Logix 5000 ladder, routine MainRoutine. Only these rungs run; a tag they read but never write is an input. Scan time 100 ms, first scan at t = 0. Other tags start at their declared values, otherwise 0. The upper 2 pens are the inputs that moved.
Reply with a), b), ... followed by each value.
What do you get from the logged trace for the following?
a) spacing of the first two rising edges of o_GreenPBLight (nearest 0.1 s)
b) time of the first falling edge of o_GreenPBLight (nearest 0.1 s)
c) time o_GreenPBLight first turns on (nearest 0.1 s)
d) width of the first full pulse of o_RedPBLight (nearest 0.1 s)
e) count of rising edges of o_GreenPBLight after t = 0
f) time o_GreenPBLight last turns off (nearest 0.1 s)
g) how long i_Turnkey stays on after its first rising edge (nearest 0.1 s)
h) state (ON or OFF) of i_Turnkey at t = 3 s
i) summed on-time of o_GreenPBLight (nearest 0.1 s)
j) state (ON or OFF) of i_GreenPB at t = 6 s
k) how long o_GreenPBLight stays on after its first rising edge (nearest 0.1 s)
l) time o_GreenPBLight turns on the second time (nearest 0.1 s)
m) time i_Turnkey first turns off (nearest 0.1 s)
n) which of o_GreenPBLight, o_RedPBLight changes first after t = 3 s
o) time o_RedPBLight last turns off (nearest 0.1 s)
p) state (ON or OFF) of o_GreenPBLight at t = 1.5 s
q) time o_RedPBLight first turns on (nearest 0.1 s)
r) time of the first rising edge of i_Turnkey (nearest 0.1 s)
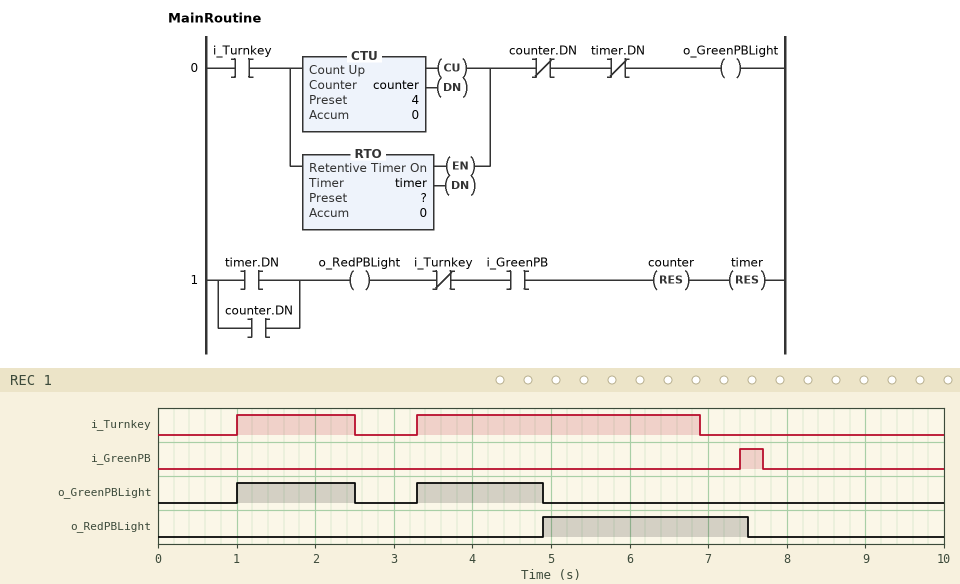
a) 2.3 s
b) 2.5 s
c) 1.0 s
d) 2.6 s
e) 2
f) 4.9 s
g) 1.5 s
h) OFF
i) 3.1 s
j) OFF
k) 1.5 s
l) 3.3 s
m) 2.5 s
n) o_GreenPBLight
o) 7.5 s
p) ON
q) 4.9 s
r) 1.0 s
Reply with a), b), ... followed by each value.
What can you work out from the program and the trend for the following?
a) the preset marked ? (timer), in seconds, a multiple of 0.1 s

a) 3.0 s
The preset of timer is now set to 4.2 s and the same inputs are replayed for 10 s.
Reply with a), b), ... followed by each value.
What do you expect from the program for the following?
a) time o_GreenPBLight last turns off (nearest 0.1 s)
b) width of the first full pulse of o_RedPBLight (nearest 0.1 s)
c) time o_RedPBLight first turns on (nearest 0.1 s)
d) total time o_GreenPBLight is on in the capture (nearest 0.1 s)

a) 6.1 s
b) 1.4 s
c) 6.1 s
d) 4.3 s
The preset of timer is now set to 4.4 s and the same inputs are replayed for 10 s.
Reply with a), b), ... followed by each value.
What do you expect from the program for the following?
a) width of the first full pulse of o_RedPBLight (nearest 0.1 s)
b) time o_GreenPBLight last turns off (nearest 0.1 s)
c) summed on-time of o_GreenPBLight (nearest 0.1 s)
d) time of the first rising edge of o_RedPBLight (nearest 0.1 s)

a) 1.2 s
b) 6.3 s
c) 4.5 s
d) 6.3 s
